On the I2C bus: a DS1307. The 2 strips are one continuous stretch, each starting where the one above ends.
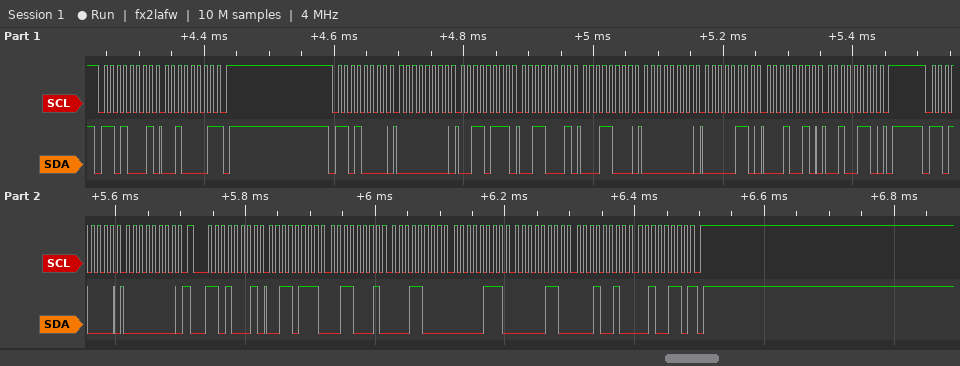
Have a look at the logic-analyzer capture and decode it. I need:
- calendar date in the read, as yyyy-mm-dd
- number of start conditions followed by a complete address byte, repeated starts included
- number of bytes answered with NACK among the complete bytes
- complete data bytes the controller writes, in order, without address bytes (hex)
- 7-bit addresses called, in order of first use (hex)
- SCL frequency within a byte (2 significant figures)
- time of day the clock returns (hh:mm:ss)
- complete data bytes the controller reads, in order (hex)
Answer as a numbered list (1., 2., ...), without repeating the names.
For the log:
1. 2026-12-06
2. 4
3. 2
4. 00 37 31 18 00 06 12 26 00
5. 0x68
6. 100 kHz
7. 18:31:37
8. 21 37 31 18 07 06 12 26
